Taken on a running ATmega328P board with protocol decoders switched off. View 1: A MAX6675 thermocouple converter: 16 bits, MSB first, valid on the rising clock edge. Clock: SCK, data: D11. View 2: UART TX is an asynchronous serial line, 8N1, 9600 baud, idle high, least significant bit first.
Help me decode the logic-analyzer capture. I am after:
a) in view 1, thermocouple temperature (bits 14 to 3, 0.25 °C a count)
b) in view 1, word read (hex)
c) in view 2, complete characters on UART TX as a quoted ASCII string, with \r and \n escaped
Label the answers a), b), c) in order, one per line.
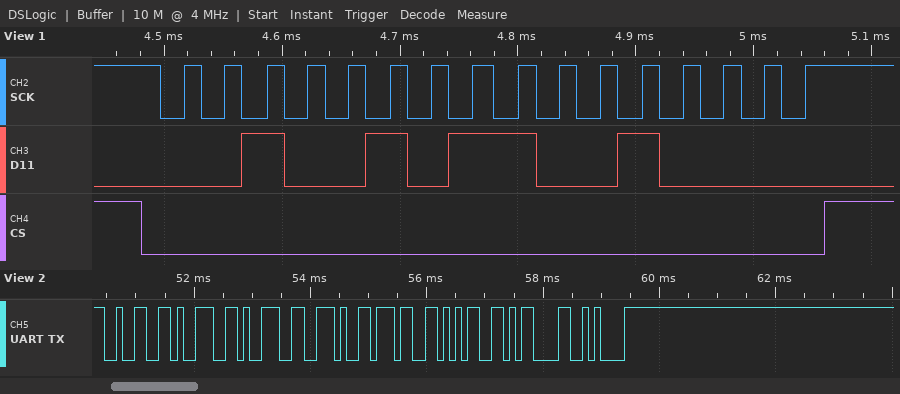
a) 300.50 °C
b) 0x2590
c) "299.75\r\n"
